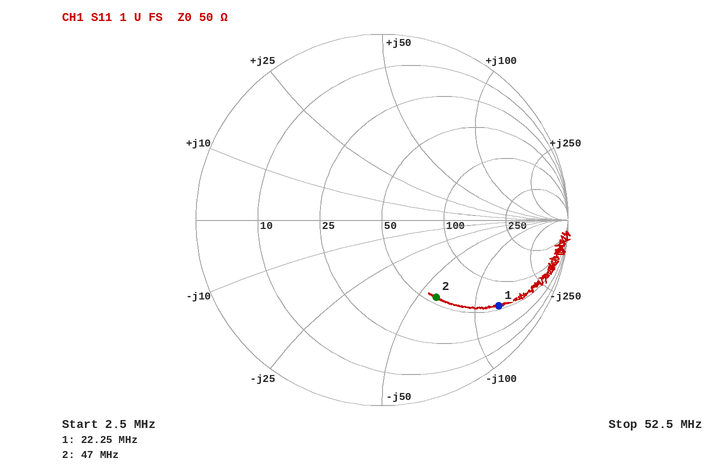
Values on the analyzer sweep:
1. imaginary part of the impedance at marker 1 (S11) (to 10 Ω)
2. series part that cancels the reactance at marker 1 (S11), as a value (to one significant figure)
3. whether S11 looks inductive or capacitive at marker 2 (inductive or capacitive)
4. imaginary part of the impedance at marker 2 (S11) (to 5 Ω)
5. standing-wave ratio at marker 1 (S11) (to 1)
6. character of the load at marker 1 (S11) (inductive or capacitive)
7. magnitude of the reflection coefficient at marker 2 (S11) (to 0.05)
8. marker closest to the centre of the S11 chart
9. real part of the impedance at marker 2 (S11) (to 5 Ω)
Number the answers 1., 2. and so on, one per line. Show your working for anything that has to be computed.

1. -130 Ω
2. L = 130 Ω/(2π × 22.25 MHz) ≈ 930 nH, so 900 nH to one significant figure
3. capacitive
4. -60 Ω
5. 8
6. capacitive
7. 0.50
8. marker 2
9. 55 Ω
